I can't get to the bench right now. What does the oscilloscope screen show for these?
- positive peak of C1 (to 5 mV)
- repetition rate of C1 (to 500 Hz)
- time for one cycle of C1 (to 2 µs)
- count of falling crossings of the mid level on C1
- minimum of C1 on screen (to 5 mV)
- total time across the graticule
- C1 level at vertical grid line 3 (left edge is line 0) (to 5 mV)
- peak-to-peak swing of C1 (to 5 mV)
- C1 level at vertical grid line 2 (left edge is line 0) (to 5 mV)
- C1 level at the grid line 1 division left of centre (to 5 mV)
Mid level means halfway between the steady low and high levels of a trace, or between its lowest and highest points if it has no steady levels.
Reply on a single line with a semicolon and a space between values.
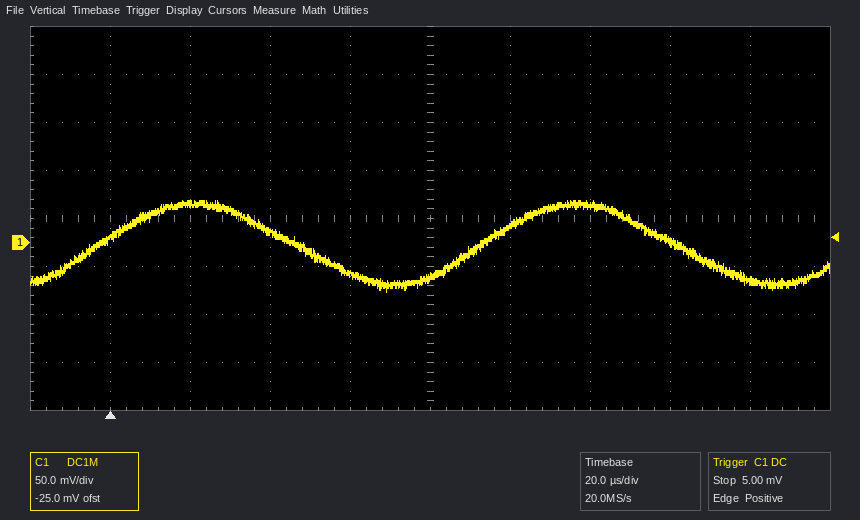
45 mV; 10.5 kHz; 96 µs; 2; -50 mV; 200 µs; 10 mV; 95 mV; 40 mV; -35 mV
